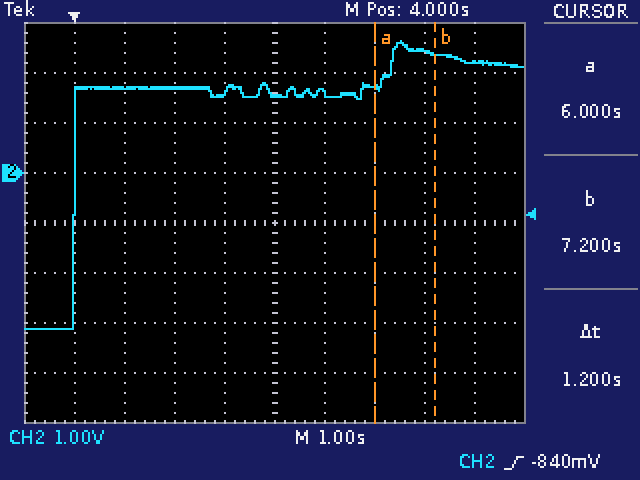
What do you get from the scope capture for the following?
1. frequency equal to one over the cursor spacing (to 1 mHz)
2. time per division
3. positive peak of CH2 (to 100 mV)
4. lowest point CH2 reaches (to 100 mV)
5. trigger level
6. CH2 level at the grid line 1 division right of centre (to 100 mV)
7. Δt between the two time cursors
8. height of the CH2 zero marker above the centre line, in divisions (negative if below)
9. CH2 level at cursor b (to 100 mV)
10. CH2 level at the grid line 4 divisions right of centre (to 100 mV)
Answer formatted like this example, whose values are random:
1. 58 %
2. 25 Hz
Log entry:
1. 833 mHz
2. 1 s
3. 2.6 V
4. -3.1 V
5. -840 mV
6. 1.6 V
7. 1.2 s
8. +1.0 div
9. 2.4 V
10. 2.2 V
